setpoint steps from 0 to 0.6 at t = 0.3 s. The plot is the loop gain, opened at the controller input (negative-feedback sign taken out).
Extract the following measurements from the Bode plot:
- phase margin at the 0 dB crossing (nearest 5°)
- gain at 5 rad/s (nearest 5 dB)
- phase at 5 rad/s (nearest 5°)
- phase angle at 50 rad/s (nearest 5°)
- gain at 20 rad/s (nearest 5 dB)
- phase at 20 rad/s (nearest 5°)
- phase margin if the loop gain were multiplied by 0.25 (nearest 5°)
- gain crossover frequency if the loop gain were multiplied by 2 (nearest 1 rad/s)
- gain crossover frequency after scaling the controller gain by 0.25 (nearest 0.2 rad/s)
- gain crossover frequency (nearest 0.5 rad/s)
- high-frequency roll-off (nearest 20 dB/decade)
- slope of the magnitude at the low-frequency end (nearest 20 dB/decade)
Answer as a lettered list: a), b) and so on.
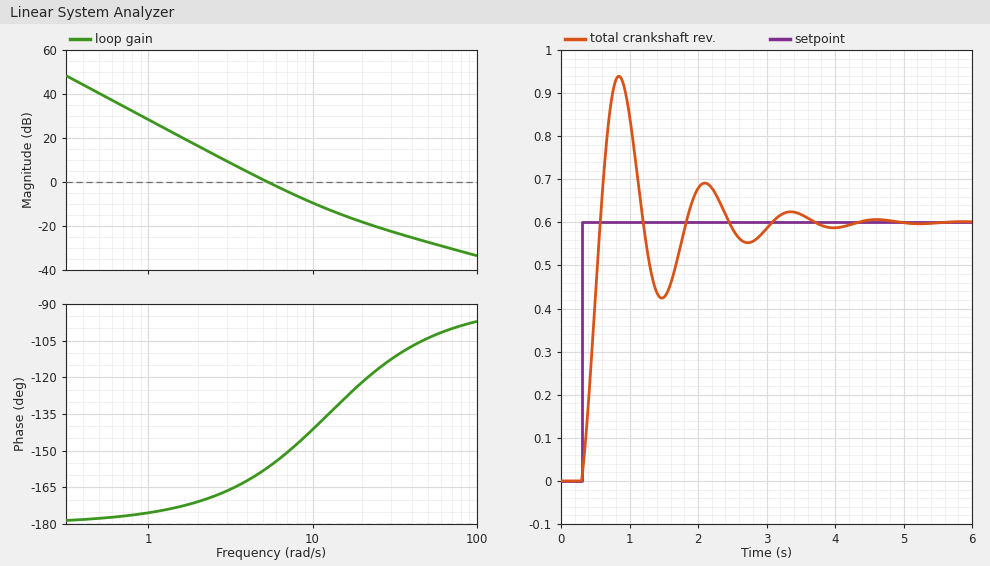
a) 25°
b) 0 dB
c) -160°
d) -105°
e) -20 dB
f) -120°
g) 10°
h) 8 rad/s
i) 2.6 rad/s
j) 5.5 rad/s
k) -20 dB/decade
l) -40 dB/decade
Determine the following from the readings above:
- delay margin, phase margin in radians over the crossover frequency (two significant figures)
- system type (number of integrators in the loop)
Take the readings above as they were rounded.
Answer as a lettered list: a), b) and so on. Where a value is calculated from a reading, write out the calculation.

a) 25 × π / 180 / 5.5 = 0.079 s
b) 2
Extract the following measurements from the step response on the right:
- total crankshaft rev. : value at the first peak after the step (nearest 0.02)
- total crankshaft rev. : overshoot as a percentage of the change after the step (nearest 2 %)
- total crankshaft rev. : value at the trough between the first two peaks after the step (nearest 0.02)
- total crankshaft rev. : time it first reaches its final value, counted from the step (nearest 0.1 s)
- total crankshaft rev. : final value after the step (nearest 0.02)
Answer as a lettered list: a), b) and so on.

a) 0.94
b) 56 %
c) 0.42
d) 0.3 s
e) 0.60
